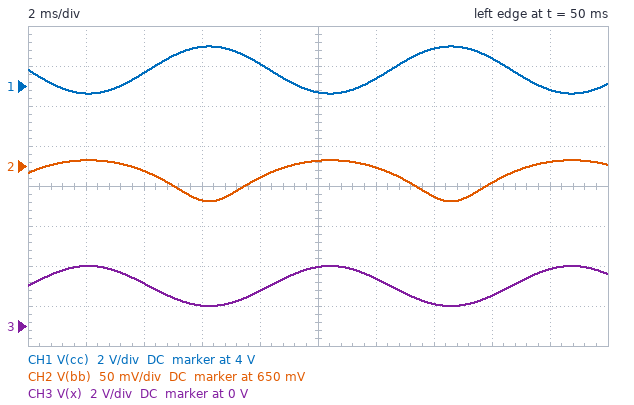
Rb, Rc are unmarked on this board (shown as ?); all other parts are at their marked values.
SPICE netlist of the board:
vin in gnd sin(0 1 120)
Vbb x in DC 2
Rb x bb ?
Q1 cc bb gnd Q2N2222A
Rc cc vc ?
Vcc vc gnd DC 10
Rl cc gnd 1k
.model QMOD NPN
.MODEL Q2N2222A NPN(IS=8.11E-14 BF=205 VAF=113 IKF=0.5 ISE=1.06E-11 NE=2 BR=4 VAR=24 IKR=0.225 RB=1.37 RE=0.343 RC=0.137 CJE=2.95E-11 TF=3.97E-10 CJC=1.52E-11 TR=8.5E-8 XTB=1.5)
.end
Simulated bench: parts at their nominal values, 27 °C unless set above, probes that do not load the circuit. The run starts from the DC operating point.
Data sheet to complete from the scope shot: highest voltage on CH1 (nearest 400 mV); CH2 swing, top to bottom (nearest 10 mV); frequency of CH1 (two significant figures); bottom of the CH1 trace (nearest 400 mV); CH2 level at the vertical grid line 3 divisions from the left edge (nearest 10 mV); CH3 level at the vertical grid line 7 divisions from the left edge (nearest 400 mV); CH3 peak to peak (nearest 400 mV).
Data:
6.0 V
50 mV
120 Hz
3.6 V
610 mV
1.2 V
2.0 V
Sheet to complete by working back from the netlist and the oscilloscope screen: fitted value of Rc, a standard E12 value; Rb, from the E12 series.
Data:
560 Ω
56 kΩ
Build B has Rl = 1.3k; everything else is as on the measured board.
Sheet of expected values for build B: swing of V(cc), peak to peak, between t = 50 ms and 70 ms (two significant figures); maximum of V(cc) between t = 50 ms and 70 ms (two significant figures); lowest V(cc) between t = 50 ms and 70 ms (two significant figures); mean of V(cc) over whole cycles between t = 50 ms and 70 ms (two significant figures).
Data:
2.6 V
6.5 V
3.9 V
5.2 V
